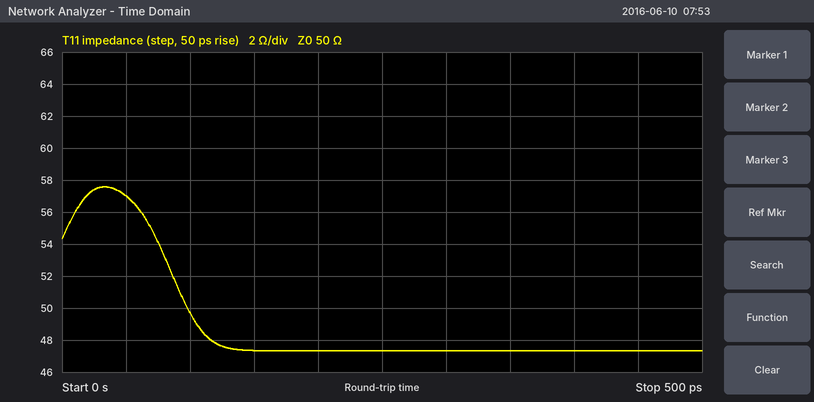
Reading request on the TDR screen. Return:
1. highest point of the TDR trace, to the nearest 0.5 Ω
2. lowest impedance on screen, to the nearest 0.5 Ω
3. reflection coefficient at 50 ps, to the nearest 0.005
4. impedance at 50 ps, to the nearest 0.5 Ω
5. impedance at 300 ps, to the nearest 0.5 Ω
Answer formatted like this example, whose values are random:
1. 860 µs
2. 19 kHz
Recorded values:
1. 57.5 Ω
2. 47.5 Ω
3. +0.065
4. 57.0 Ω
5. 47.5 Ω
